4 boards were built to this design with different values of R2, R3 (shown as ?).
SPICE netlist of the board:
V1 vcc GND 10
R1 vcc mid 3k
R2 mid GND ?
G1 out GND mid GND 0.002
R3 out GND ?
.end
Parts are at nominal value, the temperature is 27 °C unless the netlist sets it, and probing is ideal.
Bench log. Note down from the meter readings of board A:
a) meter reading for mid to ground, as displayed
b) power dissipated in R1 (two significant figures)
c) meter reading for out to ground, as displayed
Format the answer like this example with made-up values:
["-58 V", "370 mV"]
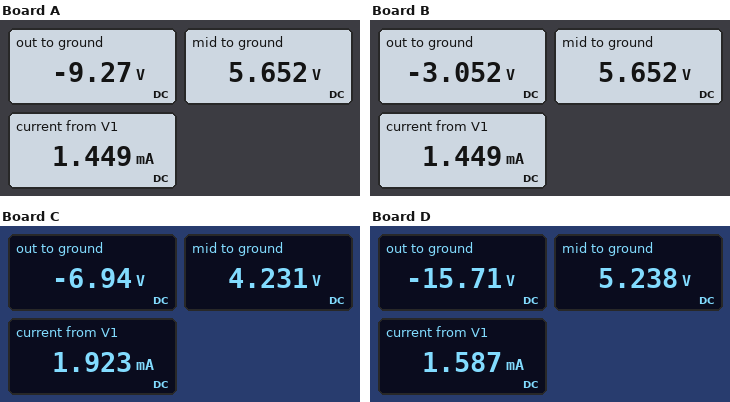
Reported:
["5.652 V", "6.3 mW", "-9.27 V"]
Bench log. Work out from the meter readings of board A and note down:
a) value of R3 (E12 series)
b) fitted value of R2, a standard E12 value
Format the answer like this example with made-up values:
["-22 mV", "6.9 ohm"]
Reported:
["820 Ω", "3.9 kΩ"]
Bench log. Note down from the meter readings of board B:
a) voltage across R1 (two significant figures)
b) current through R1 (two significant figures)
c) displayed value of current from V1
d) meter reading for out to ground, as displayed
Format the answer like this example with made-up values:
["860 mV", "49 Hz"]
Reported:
["4.3 V", "1.4 mA", "1.449 mA", "-3.052 V"]
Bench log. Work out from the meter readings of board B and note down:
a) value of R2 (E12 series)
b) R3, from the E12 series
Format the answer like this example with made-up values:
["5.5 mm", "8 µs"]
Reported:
["3.9 kΩ", "270 Ω"]
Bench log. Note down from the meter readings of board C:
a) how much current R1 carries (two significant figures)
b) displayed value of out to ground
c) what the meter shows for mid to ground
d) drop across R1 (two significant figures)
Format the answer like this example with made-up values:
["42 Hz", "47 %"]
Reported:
["1.9 mA", "-6.94 V", "4.231 V", "5.8 V"]
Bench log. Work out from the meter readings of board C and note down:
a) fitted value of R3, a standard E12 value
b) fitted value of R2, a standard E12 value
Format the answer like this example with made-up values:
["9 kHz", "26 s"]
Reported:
["820 Ω", "2.2 kΩ"]
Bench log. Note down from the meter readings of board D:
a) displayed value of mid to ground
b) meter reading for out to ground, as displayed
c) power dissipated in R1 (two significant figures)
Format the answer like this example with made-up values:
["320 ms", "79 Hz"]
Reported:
["5.238 V", "-15.71 V", "7.6 mW"]
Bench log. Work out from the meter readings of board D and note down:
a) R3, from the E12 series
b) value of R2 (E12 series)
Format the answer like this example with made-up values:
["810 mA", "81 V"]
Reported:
["1.5 kΩ", "3.3 kΩ"]
